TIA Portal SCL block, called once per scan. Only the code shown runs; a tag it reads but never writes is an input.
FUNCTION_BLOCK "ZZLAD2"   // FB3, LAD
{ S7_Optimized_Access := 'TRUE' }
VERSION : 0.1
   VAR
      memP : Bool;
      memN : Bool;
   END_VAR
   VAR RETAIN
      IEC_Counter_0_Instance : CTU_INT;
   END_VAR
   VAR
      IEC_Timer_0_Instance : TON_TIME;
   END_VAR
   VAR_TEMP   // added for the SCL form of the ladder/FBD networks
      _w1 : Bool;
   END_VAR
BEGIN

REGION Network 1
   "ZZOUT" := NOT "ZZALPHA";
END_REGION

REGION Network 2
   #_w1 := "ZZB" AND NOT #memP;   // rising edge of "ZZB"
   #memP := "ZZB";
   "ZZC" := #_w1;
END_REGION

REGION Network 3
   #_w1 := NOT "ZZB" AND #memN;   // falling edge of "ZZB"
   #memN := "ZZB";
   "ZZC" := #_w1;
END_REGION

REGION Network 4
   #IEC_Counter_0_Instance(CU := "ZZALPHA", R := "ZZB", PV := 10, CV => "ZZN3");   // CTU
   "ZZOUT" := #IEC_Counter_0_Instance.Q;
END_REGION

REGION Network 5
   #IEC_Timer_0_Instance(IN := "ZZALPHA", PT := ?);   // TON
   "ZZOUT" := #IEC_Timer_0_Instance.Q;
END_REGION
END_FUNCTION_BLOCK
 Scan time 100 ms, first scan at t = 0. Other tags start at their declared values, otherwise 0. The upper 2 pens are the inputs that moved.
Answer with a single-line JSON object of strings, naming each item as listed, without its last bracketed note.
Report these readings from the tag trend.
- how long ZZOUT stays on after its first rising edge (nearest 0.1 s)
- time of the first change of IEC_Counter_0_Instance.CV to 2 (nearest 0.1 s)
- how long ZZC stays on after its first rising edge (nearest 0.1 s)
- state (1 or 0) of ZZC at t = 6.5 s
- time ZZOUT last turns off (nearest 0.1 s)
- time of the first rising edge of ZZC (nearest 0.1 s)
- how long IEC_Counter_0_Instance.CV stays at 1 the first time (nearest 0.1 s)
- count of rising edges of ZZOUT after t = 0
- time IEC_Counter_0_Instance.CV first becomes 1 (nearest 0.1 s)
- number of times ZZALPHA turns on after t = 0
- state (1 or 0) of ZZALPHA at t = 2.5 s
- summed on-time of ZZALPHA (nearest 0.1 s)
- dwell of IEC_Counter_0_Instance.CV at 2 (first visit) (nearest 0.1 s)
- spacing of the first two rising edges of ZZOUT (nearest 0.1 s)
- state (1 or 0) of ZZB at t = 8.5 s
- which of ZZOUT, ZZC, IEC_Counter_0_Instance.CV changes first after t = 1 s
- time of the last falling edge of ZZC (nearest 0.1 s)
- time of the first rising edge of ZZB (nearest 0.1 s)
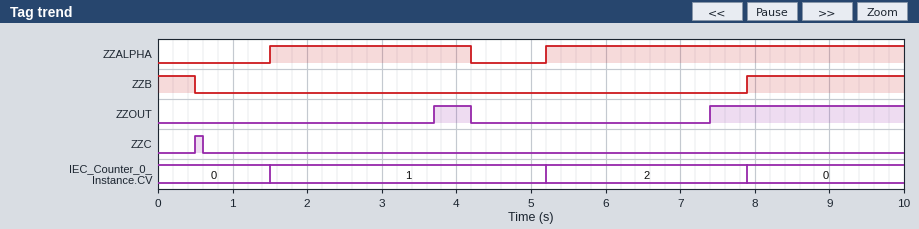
{"how long ZZOUT stays on after its first rising edge": "0.5 s", "time of the first change of IEC_Counter_0_Instance.CV to 2": "5.2 s", "how long ZZC stays on after its first rising edge": "0.1 s", "state (1 or 0) of ZZC at t = 6.5 s": "0", "time ZZOUT last turns off": "4.2 s", "time of the first rising edge of ZZC": "0.5 s", "how long IEC_Counter_0_Instance.CV stays at 1 the first time": "3.7 s", "count of rising edges of ZZOUT after t = 0": "2", "time IEC_Counter_0_Instance.CV first becomes 1": "1.5 s", "number of times ZZALPHA turns on after t = 0": "2", "state (1 or 0) of ZZALPHA at t = 2.5 s": "1", "summed on-time of ZZALPHA": "7.5 s", "dwell of IEC_Counter_0_Instance.CV at 2 (first visit)": "2.7 s", "spacing of the first two rising edges of ZZOUT": "3.7 s", "state (1 or 0) of ZZB at t = 8.5 s": "1", "which of ZZOUT, ZZC, IEC_Counter_0_Instance.CV changes first after t = 1 s": "IEC_Counter_0_Instance.CV", "time of the last falling edge of ZZC": "0.6 s", "time of the first rising edge of ZZB": "7.9 s"}
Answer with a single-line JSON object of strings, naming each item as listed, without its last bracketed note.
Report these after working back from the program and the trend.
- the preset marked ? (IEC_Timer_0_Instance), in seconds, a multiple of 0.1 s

{"the preset marked ? (IEC_Timer_0_Instance), in seconds, a multiple of 0.1 s": "2.2 s"}
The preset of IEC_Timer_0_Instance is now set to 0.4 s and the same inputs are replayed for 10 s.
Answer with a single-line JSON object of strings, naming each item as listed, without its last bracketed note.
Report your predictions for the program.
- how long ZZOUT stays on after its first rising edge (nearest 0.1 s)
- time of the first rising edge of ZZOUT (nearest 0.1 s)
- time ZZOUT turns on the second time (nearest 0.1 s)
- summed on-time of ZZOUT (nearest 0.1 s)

{"how long ZZOUT stays on after its first rising edge": "2.3 s", "time of the first rising edge of ZZOUT": "1.9 s", "time ZZOUT turns on the second time": "5.6 s", "summed on-time of ZZOUT": "6.7 s"}
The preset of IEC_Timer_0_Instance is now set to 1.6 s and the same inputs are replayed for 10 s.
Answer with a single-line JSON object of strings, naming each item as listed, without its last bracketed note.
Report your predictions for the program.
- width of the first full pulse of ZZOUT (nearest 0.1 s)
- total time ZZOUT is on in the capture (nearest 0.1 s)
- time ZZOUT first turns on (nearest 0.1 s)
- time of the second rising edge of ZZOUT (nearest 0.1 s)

{"width of the first full pulse of ZZOUT": "1.1 s", "total time ZZOUT is on in the capture": "4.3 s", "time ZZOUT first turns on": "3.1 s", "time of the second rising edge of ZZOUT": "6.8 s"}
